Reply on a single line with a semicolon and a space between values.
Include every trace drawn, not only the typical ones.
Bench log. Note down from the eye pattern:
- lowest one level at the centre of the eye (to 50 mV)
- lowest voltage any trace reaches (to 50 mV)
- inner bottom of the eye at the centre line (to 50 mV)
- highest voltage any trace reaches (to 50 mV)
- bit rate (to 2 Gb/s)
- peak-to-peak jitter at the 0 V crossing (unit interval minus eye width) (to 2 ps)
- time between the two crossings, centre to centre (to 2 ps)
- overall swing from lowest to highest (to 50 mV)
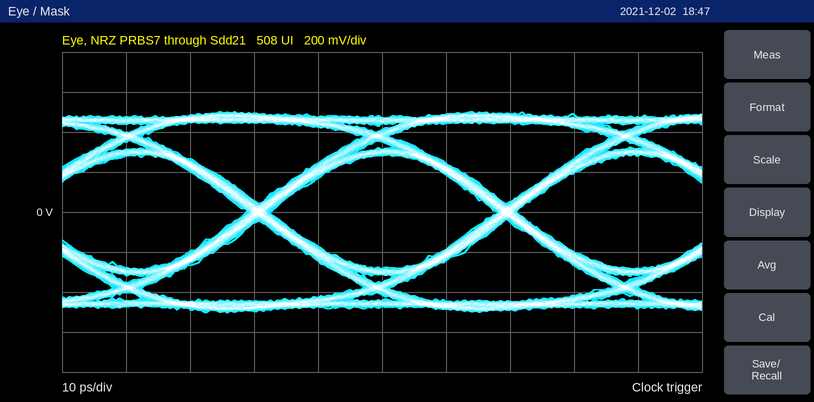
300 mV; -500 mV; -300 mV; 500 mV; 26 Gb/s; 4 ps; 38 ps; 1.00 V
